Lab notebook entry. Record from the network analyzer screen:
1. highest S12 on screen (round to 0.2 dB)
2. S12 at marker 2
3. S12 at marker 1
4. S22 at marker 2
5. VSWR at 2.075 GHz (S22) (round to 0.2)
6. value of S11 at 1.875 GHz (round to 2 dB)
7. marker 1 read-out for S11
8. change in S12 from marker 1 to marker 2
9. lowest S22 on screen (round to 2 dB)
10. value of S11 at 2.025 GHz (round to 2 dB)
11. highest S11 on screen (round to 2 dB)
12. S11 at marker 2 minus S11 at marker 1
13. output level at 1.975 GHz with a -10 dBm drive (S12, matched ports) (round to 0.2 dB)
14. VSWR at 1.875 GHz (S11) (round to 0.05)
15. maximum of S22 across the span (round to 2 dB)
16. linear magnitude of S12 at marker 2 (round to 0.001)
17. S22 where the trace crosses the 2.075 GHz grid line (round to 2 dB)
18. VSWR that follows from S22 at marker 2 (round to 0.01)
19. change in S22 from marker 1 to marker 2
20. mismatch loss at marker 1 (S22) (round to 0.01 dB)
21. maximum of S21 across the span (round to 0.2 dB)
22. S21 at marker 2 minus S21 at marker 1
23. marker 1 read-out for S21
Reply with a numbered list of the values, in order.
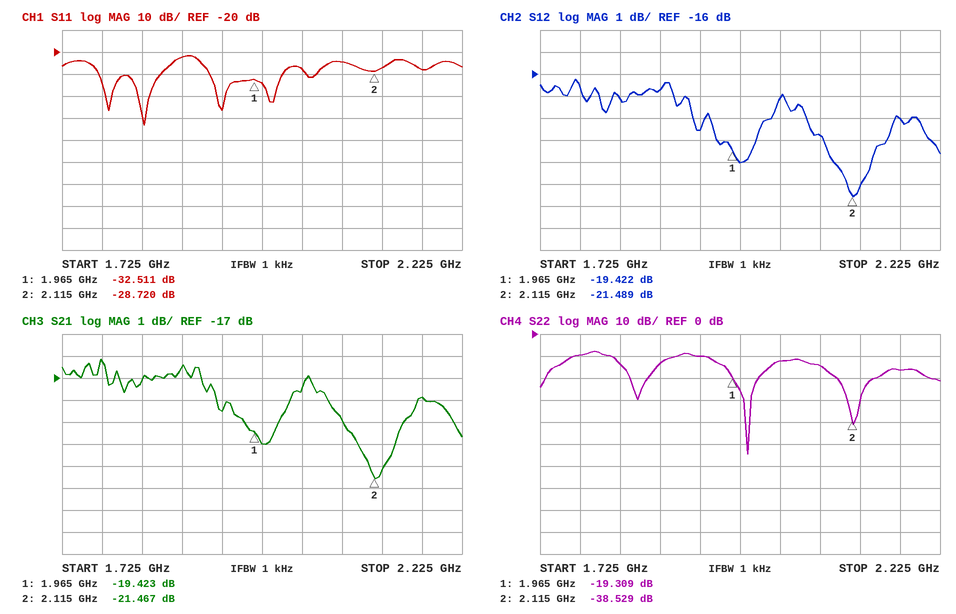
1. -16.2 dB
2. -21.489 dB
3. -19.422 dB
4. -38.529 dB
5. 1.4
6. -22 dB
7. -32.511 dB
8. -2.067 dB
9. -54 dB
10. -28 dB
11. -22 dB
12. 3.791 dB
13. -30.0 dBm
14. 1.15
15. -8 dB
16. 0.084
17. -14 dB
18. 1.02
19. -19.220 dB
20. 0.05 dB
21. -16.2 dB
22. -2.044 dB
23. -19.423 dB
